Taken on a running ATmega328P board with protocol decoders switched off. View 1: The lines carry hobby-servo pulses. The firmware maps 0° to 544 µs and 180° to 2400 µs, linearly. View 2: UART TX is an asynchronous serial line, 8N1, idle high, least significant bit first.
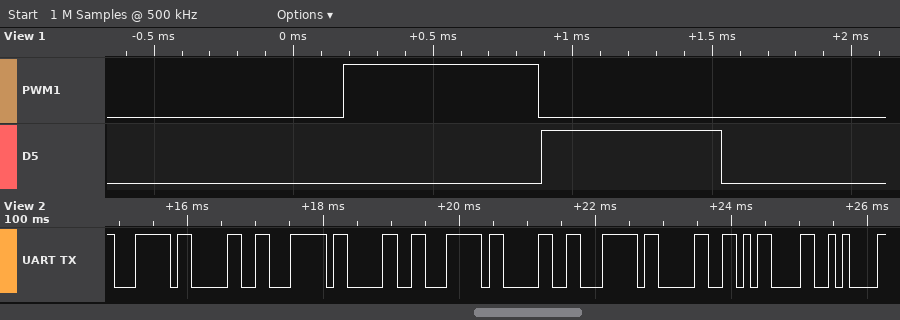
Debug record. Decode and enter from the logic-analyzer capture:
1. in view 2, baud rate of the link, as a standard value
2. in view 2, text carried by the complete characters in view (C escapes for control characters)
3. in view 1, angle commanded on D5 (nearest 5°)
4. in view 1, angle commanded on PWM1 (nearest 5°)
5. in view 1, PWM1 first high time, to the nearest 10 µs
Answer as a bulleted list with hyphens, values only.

- 9600 baud
- "|0|0|0|0\r\n"
- 10°
- 15°
- 700 µs
